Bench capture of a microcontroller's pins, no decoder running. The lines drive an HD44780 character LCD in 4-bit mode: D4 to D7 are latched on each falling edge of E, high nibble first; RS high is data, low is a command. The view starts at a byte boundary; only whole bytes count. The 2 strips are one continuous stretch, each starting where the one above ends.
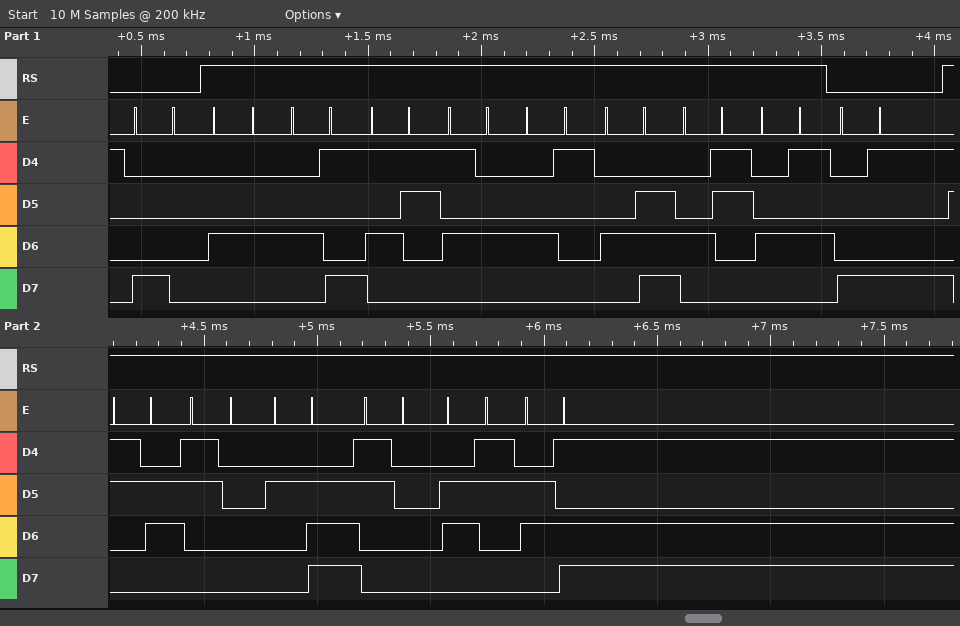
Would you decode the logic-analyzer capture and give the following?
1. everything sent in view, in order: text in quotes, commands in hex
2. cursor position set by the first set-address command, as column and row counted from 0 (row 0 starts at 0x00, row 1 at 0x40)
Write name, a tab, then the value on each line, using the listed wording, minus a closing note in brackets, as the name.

everything sent in view, in order: text in quotes, commands in hex	0x80 "DISTANCE" 0x89 "60.0cm"
cursor position set by the first set-address command, as column and row counted from 0	column 0, row 0
